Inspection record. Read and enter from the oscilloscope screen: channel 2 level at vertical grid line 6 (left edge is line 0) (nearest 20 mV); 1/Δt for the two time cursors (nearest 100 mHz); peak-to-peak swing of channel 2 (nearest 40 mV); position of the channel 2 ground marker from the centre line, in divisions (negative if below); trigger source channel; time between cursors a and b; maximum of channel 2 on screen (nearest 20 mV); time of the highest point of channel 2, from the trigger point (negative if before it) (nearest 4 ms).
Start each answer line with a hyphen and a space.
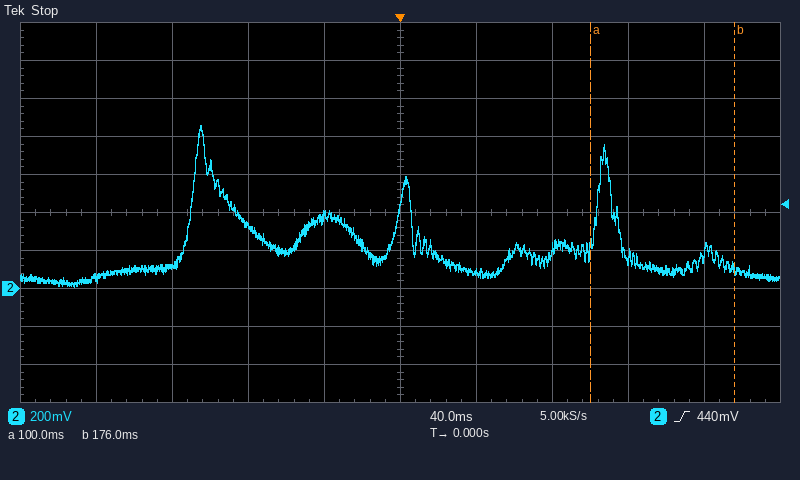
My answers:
- 80 mV
- 13.2 Hz
- 840 mV
- -2.0 div
- channel 2
- 76 ms
- 860 mV
- -104 ms
